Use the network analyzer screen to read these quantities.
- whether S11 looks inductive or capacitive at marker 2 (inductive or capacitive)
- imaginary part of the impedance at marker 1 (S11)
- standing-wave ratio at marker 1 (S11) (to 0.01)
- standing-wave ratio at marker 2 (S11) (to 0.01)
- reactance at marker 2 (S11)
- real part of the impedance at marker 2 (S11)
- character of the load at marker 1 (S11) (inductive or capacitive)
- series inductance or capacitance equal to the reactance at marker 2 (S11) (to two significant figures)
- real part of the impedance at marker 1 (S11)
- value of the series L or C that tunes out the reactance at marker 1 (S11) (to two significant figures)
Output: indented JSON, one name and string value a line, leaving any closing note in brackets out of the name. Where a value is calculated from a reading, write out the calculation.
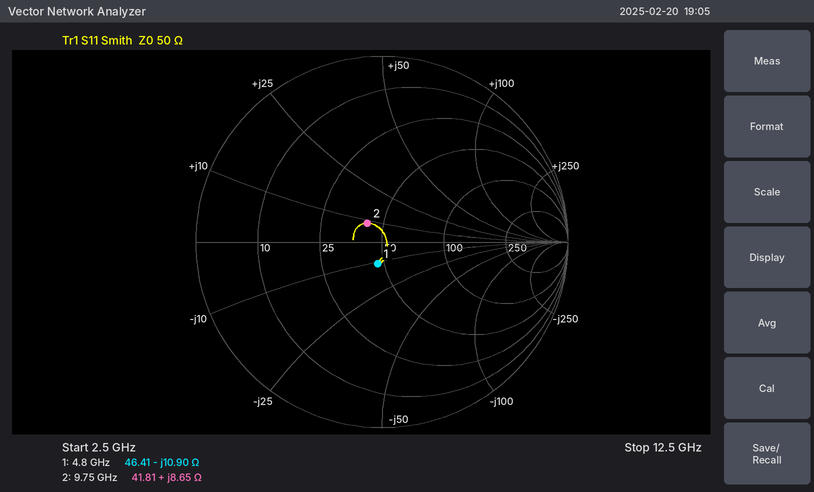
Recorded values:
{
  "whether S11 looks inductive or capacitive at marker 2": "inductive",
  "imaginary part of the impedance at marker 1": "-10.90 Ω",
  "standing-wave ratio at marker 1 (S11)": "1.27",
  "standing-wave ratio at marker 2 (S11)": "1.30",
  "reactance at marker 2": "+8.65 Ω",
  "real part of the impedance at marker 2": "41.81 Ω",
  "character of the load at marker 1 (S11)": "capacitive",
  "series inductance or capacitance equal to the reactance at marker 2 (S11)": "L = 8.65 Ω/(2π × 9.75 GHz) ≈ 141 pH, so 140 pH to two significant figures",
  "real part of the impedance at marker 1": "46.41 Ω",
  "value of the series L or C that tunes out the reactance at marker 1 (S11)": "L = 10.9 Ω/(2π × 4.8 GHz) ≈ 361 pH, so 360 pH to two significant figures"
}
